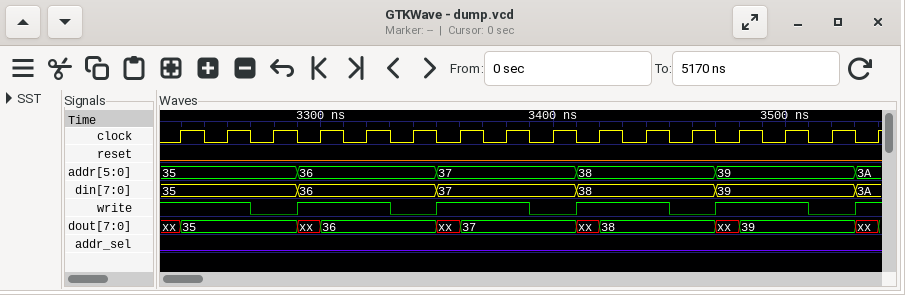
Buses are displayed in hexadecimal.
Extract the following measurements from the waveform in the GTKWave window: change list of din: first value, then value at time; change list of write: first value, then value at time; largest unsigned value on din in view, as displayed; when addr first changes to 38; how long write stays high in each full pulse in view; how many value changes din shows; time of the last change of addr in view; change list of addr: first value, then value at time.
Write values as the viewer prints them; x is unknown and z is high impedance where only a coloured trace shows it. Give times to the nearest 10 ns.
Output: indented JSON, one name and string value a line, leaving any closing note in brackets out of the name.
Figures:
{
  "change list of din: first value, then value at time": "35, 36 at 3290 ns, 37 at 3350 ns, 38 at 3410 ns, 39 at 3470 ns, 3A at 3530 ns",
  "change list of write: first value, then value at time": "1, 0 at 3270 ns, 1 at 3290 ns, 0 at 3330 ns, 1 at 3350 ns, 0 at 3390 ns, 1 at 3410 ns, 0 at 3450 ns, 1 at 3470 ns, 0 at 3510 ns, 1 at 3530 ns",
  "largest unsigned value on din in view, as displayed": "3A",
  "when addr first changes to 38": "3410 ns",
  "how long write stays high in each full pulse in view": "40 ns, 40 ns, 40 ns, 40 ns",
  "how many value changes din shows": "5",
  "time of the last change of addr in view": "3530 ns",
  "change list of addr: first value, then value at time": "35, 36 at 3290 ns, 37 at 3350 ns, 38 at 3410 ns, 39 at 3470 ns, 3A at 3530 ns"
}
